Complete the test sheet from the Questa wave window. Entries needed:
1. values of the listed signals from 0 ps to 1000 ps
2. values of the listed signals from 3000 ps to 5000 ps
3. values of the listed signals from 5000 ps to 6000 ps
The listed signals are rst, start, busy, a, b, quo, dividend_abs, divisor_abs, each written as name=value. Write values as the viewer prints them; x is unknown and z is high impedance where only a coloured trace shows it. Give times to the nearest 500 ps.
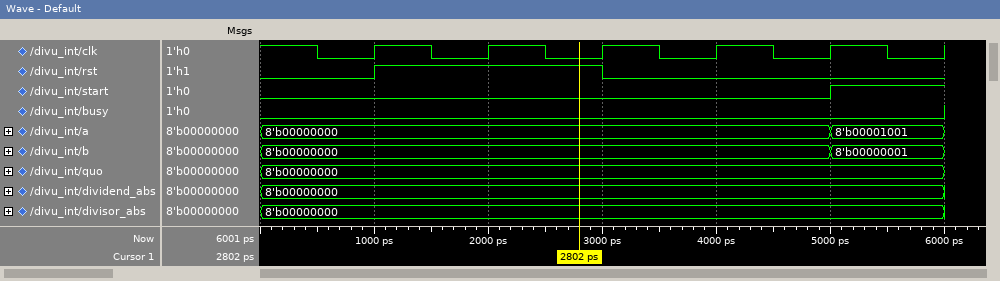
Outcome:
rst=0, start=0, busy=0, a=8'b00000000, b=8'b00000000, quo=8'b00000000, dividend_abs=8'b00000000, divisor_abs=8'b00000000
rst=0, start=0, busy=0, a=8'b00000000, b=8'b00000000, quo=8'b00000000, dividend_abs=8'b00000000, divisor_abs=8'b00000000
rst=0, start=1, busy=0, a=8'b00001001, b=8'b00000001, quo=8'b00000000, dividend_abs=8'b00000000, divisor_abs=8'b00000000
